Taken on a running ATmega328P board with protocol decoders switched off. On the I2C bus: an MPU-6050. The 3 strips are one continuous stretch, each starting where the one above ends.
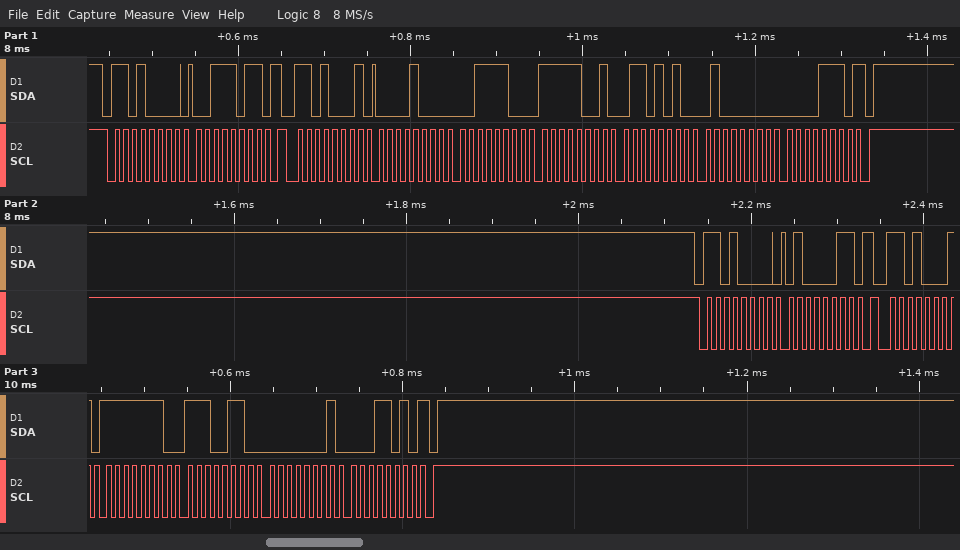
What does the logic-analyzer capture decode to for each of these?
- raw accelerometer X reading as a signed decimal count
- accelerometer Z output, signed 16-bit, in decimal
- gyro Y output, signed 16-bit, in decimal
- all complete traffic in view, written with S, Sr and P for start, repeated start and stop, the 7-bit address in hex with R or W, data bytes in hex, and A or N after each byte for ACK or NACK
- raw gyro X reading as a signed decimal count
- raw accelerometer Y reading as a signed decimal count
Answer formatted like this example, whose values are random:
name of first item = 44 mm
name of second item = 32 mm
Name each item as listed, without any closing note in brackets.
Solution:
raw accelerometer X reading as a signed decimal count = 2108
accelerometer Z output, signed 16-bit, in decimal = 16398
gyro Y output, signed 16-bit, in decimal = 282
all complete traffic in view, written with S, Sr and P for start, repeated start and stop, the 7-bit address in hex with R or W, data bytes in hex, and A or N after each byte for ACK or NACK = S 68W A 3B A Sr 68R A 08 A 3C A F9 A 6A A 40 A 0E N P S 68W A 43 A Sr 68R A FE A E6 A 01 A 1A N P
raw gyro X reading as a signed decimal count = -282
raw accelerometer Y reading as a signed decimal count = -1686
